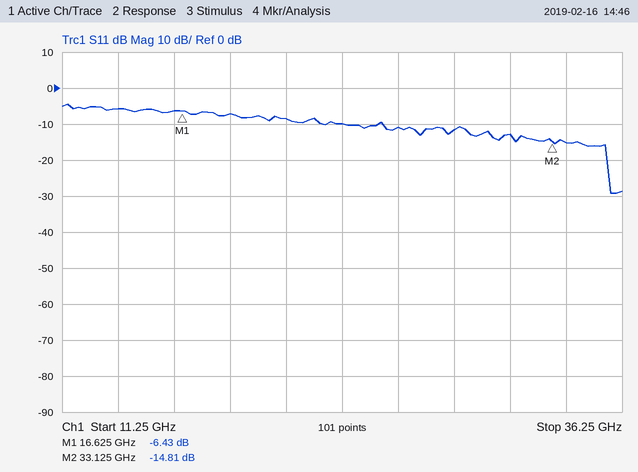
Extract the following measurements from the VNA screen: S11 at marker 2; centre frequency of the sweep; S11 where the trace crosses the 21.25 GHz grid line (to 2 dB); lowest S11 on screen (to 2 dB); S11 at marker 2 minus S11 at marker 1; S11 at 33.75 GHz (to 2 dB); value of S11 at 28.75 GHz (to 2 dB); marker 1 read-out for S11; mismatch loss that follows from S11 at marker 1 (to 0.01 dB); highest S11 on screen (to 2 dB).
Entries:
-14.81 dB
23.75 GHz
-8 dB
-30 dB
-8.38 dB
-16 dB
-12 dB
-6.43 dB
1.12 dB
-4 dB
